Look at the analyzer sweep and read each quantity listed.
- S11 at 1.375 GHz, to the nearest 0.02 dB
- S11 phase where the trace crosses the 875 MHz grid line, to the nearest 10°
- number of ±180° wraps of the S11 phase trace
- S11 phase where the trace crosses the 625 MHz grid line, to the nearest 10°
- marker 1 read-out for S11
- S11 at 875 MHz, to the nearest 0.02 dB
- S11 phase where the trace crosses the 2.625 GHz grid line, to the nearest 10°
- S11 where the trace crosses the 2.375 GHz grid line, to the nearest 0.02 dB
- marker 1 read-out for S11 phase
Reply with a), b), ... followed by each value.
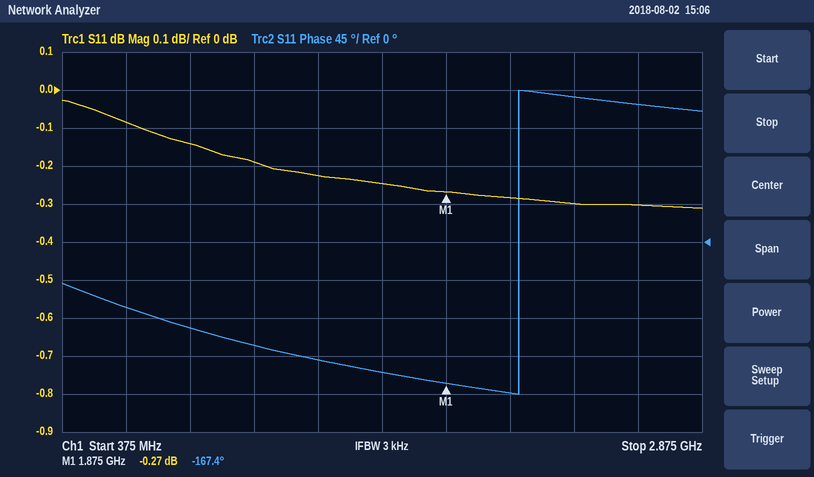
a) -0.22 dB
b) -100°
c) 1
d) -80°
e) -0.27 dB
f) -0.14 dB
g) 160°
h) -0.30 dB
i) -167.4°
